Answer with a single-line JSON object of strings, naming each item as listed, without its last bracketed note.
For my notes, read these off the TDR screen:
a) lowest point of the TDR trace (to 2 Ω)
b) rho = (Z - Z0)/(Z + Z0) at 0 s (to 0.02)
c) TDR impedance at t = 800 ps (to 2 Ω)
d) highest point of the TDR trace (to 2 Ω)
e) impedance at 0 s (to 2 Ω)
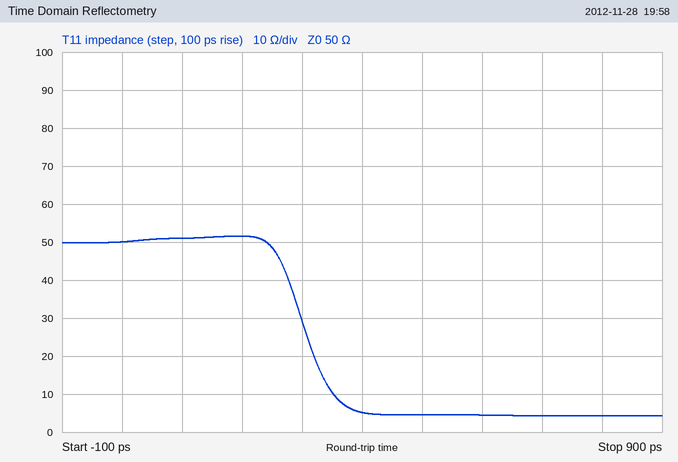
{"lowest point of the TDR trace": "4 Ω", "rho = (Z - Z0)/(Z + Z0) at 0 s": "0.00", "TDR impedance at t = 800 ps": "4 Ω", "highest point of the TDR trace": "52 Ω", "impedance at 0 s": "50 Ω"}
